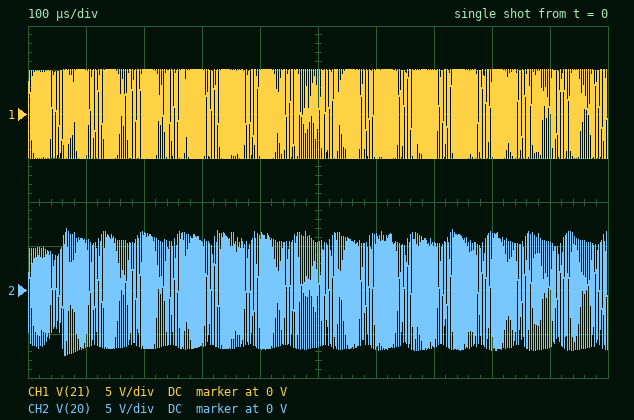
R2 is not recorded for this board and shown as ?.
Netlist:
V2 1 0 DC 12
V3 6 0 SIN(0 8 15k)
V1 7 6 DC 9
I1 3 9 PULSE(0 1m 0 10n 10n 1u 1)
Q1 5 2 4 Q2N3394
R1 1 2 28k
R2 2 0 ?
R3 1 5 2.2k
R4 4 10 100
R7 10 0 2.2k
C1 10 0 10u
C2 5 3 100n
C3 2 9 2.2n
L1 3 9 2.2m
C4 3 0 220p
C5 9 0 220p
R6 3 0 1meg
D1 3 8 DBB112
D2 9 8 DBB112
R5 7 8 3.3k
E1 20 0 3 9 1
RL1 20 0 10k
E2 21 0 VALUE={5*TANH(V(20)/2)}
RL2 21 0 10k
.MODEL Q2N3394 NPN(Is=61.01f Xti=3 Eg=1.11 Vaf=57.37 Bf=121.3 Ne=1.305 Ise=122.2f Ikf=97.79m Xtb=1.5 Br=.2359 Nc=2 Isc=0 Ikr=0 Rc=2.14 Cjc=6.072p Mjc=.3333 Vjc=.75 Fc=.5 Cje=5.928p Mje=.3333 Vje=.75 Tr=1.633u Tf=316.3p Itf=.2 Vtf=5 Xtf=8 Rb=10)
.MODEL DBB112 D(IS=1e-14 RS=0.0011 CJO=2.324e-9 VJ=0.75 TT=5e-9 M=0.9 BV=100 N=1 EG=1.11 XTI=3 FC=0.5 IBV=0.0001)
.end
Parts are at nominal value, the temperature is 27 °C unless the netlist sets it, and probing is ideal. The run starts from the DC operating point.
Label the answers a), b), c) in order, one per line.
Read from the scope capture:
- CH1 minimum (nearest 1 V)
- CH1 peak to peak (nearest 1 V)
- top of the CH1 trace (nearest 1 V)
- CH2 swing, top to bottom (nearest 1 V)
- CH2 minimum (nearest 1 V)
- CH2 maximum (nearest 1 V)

a) -5 V
b) 10 V
c) 5 V
d) 14 V
e) -7 V
f) 7 V
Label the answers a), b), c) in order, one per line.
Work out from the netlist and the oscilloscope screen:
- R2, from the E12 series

a) 4.7 kΩ
